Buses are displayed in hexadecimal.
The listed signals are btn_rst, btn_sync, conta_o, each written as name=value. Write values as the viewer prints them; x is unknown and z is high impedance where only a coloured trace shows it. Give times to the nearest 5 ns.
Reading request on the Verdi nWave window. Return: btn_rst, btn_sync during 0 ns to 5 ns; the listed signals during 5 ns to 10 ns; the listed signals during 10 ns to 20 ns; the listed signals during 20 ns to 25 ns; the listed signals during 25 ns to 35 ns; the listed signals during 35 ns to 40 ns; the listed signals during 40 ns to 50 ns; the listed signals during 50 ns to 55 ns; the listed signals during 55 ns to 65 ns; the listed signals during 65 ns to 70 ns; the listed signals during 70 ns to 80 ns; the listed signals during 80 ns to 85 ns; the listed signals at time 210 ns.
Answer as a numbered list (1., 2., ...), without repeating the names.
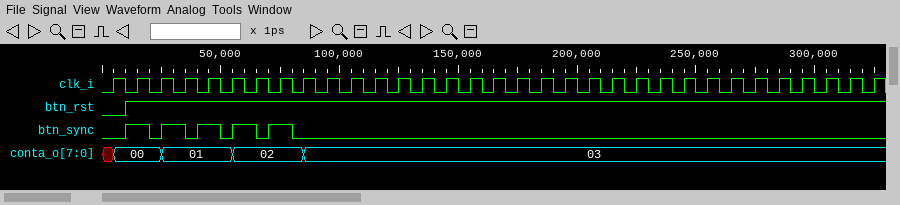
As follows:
1. btn_rst=0, btn_sync=0
2. btn_rst=0, btn_sync=0, conta_o=00
3. btn_rst=1, btn_sync=1, conta_o=00
4. btn_rst=1, btn_sync=0, conta_o=00
5. btn_rst=1, btn_sync=1, conta_o=01
6. btn_rst=1, btn_sync=0, conta_o=01
7. btn_rst=1, btn_sync=1, conta_o=01
8. btn_rst=1, btn_sync=0, conta_o=01
9. btn_rst=1, btn_sync=1, conta_o=02
10. btn_rst=1, btn_sync=0, conta_o=02
11. btn_rst=1, btn_sync=1, conta_o=02
12. btn_rst=1, btn_sync=0, conta_o=02
13. btn_rst=1, btn_sync=0, conta_o=03
